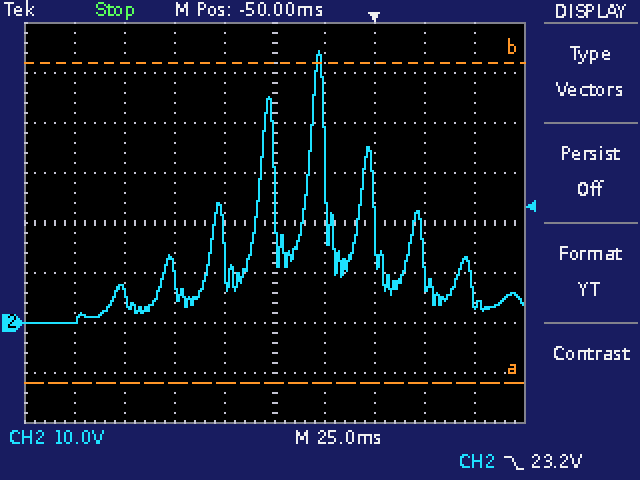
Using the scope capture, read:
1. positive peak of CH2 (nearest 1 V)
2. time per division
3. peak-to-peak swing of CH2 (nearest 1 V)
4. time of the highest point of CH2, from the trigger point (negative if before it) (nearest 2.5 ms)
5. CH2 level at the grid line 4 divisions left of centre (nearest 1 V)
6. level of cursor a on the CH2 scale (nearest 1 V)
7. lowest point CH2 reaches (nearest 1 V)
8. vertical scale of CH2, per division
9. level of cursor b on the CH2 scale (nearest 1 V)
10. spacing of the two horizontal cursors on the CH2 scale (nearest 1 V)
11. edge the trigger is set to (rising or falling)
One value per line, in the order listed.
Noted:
54 V
25 ms
54 V
-27.5 ms
1 V
-12 V
0 V
10 V
52 V
64 V
falling
